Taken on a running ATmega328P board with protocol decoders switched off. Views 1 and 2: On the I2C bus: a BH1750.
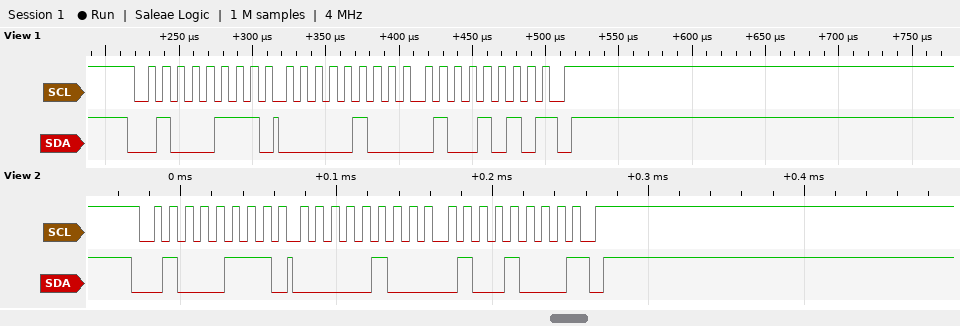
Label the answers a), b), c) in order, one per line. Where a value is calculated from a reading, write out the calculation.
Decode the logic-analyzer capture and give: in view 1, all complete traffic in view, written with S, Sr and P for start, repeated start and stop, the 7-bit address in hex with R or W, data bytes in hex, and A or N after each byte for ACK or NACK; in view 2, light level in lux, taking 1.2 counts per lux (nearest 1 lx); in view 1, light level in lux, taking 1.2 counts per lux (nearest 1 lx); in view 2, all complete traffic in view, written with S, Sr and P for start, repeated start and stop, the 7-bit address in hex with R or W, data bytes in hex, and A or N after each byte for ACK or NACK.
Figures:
a) S 23R A 04 A 4A N P
b) 1096 / 1.2 = 913 lx
c) 1098 / 1.2 = 915 lx
d) S 23R A 04 A 48 N P
